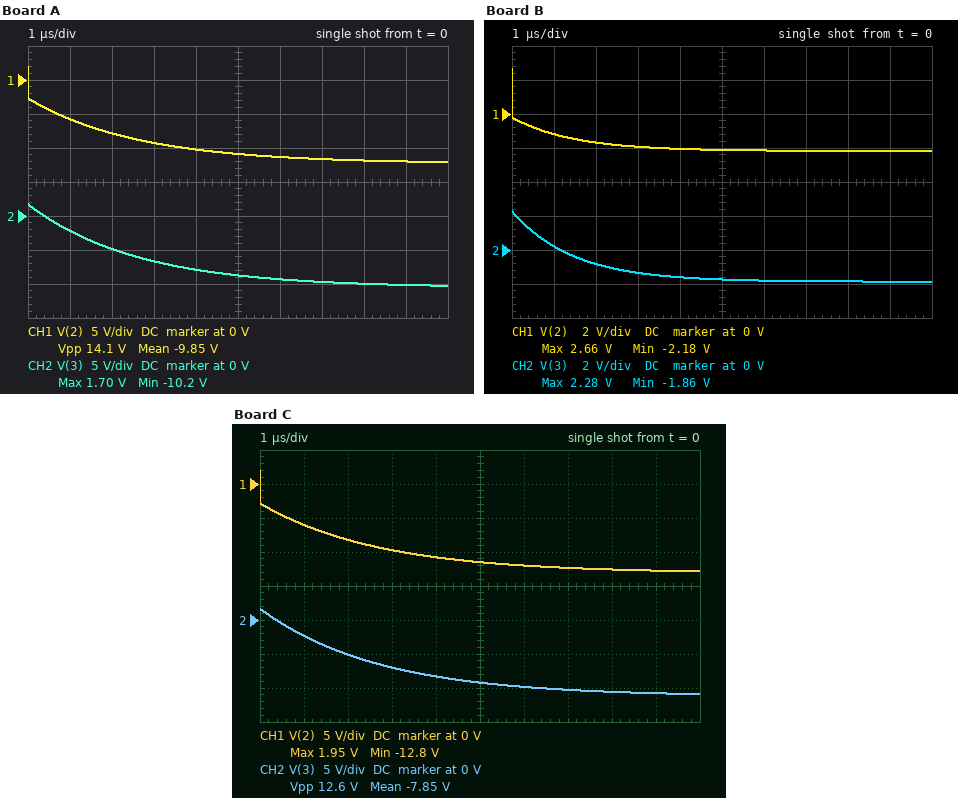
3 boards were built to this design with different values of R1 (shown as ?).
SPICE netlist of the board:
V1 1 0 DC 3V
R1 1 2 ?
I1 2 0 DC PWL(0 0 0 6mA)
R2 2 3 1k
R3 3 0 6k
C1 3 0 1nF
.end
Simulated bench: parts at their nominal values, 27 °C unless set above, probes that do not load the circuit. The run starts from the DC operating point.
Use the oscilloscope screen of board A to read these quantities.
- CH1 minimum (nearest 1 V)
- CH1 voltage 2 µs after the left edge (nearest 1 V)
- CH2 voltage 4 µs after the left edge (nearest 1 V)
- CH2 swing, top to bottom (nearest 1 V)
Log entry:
-12 V
-8 V
-8 V
12 V
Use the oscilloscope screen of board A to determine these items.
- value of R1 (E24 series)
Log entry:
3.6 kΩ
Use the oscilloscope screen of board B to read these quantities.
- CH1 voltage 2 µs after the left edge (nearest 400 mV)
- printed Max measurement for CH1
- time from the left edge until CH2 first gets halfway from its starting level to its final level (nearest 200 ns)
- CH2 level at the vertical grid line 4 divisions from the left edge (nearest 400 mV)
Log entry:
-1.6 V
2.66 V
1.0 µs
-1.6 V
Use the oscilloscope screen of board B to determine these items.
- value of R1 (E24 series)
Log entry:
910 Ω
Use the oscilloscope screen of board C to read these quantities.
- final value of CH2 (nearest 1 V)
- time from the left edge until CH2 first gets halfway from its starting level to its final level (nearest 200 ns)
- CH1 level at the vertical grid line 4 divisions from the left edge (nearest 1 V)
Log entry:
-11 V
1.8 µs
-11 V
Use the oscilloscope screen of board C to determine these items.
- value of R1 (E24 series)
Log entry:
3.9 kΩ
